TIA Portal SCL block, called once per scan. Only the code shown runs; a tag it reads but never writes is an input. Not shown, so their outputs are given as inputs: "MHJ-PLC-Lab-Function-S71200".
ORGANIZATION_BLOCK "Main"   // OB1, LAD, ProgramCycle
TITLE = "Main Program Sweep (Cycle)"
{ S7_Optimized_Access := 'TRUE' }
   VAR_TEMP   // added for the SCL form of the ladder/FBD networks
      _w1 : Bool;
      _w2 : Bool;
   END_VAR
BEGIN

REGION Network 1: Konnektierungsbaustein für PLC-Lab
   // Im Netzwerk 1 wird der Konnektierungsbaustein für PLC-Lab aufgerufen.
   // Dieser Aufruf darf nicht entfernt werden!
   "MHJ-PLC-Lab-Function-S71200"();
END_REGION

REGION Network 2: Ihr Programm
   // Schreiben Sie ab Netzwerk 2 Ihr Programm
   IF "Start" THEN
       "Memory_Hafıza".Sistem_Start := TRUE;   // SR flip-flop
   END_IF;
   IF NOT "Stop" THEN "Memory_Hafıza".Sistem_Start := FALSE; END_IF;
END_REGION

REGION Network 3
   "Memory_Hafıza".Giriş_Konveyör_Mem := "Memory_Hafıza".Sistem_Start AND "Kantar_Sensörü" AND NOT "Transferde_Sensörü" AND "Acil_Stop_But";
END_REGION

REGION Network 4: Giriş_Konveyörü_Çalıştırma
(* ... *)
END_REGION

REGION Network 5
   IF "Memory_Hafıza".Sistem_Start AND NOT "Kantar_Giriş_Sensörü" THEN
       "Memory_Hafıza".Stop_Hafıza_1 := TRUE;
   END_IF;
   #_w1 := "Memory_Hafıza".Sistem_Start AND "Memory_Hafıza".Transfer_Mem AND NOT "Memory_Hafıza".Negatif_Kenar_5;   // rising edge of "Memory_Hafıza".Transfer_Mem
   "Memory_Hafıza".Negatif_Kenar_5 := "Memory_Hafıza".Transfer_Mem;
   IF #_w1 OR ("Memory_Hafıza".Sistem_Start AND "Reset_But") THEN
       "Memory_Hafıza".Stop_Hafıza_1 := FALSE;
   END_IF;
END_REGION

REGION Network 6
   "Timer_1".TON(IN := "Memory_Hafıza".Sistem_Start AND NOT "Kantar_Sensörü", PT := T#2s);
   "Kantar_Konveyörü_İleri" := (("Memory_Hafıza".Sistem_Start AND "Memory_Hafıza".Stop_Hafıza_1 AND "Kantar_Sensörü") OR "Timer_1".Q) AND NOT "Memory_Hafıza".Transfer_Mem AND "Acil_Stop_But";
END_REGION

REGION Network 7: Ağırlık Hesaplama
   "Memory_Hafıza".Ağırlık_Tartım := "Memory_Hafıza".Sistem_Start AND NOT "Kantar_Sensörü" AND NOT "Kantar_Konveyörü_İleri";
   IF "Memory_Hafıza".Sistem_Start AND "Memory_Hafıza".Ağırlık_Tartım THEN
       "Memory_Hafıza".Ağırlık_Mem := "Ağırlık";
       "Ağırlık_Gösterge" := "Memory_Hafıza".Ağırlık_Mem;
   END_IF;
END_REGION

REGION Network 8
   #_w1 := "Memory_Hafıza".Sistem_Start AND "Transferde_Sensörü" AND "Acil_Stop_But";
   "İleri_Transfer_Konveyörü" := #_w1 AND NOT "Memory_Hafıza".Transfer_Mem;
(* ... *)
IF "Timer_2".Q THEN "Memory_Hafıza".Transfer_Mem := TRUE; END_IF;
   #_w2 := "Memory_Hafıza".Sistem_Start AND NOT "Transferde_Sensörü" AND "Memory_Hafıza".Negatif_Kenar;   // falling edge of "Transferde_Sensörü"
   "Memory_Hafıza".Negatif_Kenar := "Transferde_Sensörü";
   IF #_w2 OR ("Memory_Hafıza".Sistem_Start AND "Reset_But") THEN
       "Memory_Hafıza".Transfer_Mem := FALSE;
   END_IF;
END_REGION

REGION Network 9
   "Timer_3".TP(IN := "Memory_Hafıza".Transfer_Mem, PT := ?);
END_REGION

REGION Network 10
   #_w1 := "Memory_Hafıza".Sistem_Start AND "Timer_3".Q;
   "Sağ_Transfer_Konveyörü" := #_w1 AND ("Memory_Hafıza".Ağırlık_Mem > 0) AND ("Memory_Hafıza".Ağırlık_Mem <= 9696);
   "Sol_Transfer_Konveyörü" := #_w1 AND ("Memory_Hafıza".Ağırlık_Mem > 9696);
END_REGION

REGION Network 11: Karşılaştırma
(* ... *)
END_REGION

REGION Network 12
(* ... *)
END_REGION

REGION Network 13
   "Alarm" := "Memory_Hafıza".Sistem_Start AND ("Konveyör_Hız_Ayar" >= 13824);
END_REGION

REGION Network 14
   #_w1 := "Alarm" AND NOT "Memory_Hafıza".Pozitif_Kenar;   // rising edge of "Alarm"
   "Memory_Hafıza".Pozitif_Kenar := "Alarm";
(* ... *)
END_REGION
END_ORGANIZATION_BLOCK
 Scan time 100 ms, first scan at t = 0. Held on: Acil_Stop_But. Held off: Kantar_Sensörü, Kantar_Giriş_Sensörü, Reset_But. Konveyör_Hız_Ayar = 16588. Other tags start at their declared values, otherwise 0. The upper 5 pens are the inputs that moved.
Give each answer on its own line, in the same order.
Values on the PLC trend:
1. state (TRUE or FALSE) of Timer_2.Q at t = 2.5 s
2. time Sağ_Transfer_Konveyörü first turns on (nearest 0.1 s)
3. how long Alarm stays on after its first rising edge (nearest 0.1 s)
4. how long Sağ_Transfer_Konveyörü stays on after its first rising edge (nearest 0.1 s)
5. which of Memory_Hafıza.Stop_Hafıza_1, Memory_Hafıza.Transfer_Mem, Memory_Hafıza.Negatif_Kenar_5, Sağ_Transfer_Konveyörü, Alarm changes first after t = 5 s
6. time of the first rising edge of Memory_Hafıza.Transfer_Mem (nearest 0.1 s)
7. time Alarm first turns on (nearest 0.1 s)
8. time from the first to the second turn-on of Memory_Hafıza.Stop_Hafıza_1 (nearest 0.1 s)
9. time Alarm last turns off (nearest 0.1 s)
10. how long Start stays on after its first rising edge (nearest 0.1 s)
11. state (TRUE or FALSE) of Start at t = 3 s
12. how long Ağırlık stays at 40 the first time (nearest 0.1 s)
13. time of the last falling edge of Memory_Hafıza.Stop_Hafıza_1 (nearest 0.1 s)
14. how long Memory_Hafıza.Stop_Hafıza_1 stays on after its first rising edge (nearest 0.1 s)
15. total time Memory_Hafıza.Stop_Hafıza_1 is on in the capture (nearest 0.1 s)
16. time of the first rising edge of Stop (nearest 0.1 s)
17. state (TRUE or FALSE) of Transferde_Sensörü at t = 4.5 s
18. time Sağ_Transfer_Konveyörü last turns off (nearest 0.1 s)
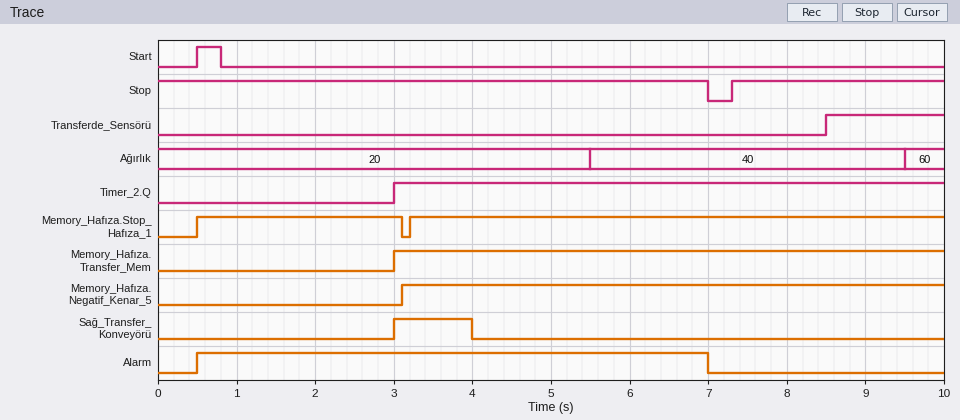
FALSE
3.0 s
6.5 s
1.0 s
Alarm
3.0 s
0.5 s
2.7 s
7.0 s
0.3 s
FALSE
4.0 s
3.1 s
2.6 s
9.4 s
7.3 s
FALSE
4.0 s
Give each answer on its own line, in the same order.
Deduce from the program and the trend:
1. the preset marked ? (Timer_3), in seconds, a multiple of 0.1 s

1.0 s
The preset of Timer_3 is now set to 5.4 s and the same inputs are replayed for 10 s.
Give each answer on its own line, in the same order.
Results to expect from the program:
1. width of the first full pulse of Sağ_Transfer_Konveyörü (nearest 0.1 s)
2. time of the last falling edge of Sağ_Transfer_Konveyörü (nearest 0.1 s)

4.0 s
7.0 s
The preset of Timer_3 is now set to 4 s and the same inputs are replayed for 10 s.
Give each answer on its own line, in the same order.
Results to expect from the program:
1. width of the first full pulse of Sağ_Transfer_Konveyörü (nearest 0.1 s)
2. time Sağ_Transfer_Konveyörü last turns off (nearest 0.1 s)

4.0 s
7.0 s
